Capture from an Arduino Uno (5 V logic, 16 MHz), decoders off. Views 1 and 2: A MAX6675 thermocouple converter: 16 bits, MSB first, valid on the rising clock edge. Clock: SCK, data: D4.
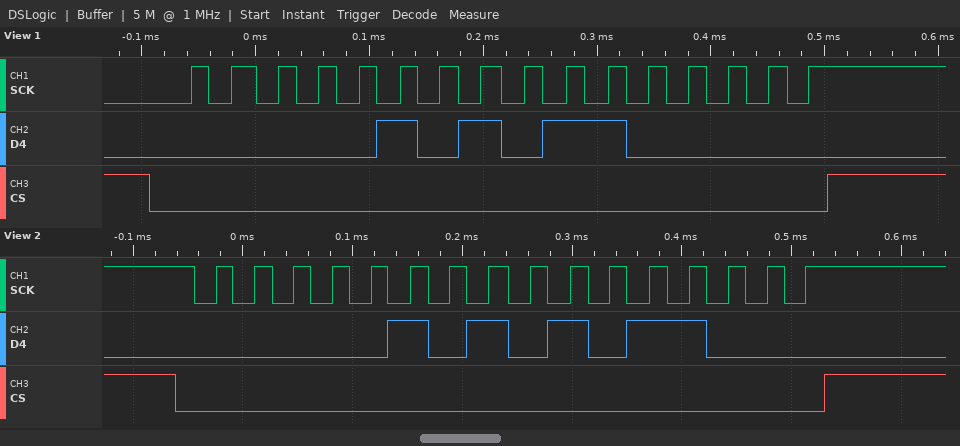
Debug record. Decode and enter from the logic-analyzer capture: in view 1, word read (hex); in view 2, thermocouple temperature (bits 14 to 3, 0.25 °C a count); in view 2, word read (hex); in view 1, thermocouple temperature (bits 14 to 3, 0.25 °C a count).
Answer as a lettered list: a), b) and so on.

a) 0x0560
b) 42.75 °C
c) 0x0558
d) 43.00 °C
